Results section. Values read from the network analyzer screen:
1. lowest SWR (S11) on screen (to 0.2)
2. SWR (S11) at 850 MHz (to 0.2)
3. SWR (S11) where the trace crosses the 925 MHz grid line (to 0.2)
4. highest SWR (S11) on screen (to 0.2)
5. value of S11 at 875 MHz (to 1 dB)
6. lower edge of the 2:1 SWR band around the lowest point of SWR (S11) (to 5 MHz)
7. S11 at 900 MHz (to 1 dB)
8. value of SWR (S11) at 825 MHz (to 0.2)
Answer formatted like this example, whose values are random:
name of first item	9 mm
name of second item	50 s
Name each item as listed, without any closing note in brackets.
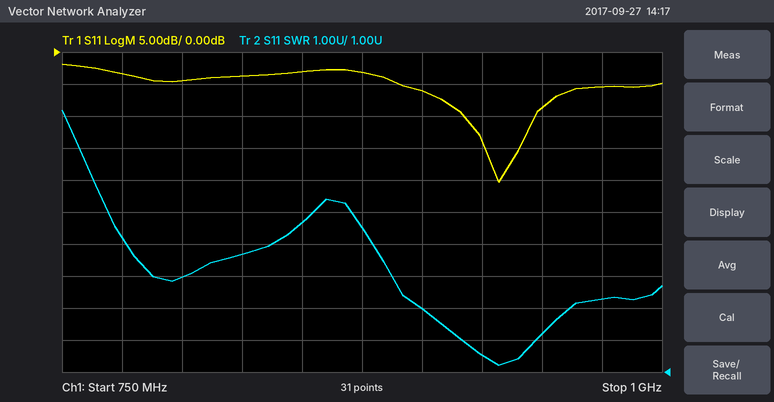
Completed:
lowest SWR (S11) on screen	1.2
SWR (S11) at 850 MHz	5.6
SWR (S11) where the trace crosses the 925 MHz grid line	1.6
highest SWR (S11) on screen	9.2
value of S11 at 875 MHz	-3 dB
lower edge of the 2:1 SWR band around the lowest point of SWR (S11)	915 MHz
S11 at 900 MHz	-6 dB
value of SWR (S11) at 825 MHz	4.6
